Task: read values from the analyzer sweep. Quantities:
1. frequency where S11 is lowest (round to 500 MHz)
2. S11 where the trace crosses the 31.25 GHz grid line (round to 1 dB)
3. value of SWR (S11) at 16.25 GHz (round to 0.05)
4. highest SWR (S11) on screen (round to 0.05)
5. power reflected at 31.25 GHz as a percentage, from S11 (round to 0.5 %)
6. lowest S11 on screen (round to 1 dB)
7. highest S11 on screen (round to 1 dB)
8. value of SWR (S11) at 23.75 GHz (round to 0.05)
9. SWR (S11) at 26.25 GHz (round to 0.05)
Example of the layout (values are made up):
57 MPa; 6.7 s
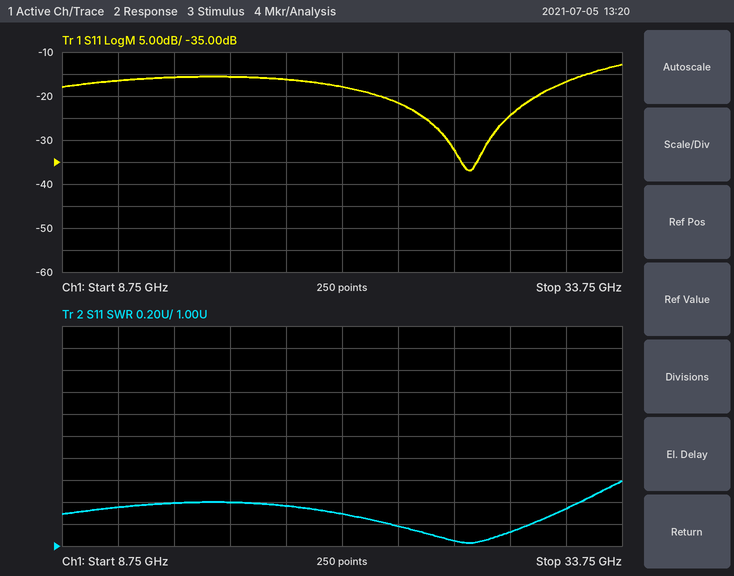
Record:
27.0 GHz; -17 dB; 1.40; 1.60; 2.0 %; -37 dB; -13 dB; 1.20; 1.05
